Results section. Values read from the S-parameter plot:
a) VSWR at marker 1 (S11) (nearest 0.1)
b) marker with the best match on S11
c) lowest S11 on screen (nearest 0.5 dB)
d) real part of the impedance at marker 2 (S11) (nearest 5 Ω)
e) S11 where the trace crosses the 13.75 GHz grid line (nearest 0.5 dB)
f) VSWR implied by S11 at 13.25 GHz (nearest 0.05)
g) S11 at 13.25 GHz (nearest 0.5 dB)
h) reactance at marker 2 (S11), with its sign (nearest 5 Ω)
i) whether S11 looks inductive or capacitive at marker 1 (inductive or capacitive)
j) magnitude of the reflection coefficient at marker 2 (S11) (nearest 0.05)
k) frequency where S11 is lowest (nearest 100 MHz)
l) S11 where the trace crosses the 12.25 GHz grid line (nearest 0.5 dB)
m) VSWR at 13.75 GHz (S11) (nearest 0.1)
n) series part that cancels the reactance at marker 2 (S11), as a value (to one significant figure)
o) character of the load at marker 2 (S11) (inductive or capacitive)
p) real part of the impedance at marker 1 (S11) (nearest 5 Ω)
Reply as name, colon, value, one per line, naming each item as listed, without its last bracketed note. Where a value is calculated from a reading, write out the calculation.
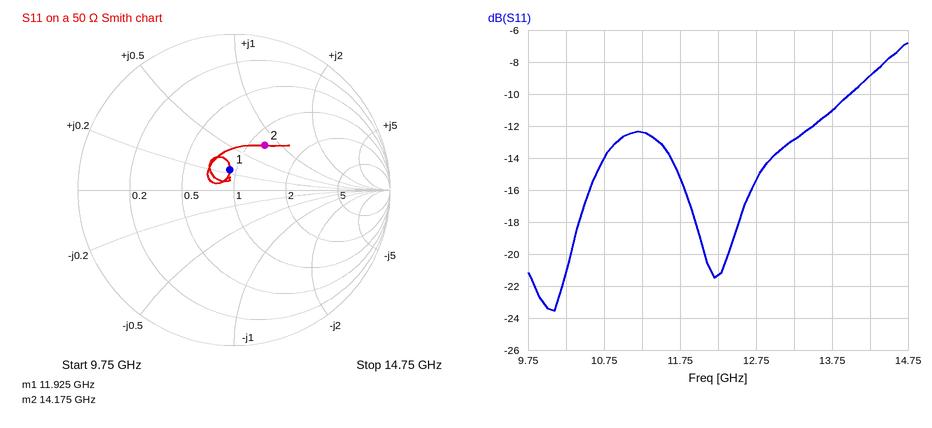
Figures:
VSWR at marker 1 (S11): 1.3
marker with the best match on S11: marker 1
lowest S11 on screen: -23.5 dB
real part of the impedance at marker 2 (S11): 60 Ω
S11 where the trace crosses the 13.75 GHz grid line: -11.0 dB
VSWR implied by S11 at 13.25 GHz: |Γ| = 10^(-13/20) = 0.2239; VSWR = (1 + 0.2239)/(1 − 0.2239) ≈ 1.58, so 1.60 to the nearest 0.05
S11 at 13.25 GHz: -13.0 dB
reactance at marker 2 (S11), with its sign: +40 Ω
whether S11 looks inductive or capacitive at marker 1: inductive
magnitude of the reflection coefficient at marker 2 (S11): 0.35
frequency where S11 is lowest: 10.1 GHz
S11 where the trace crosses the 12.25 GHz grid line: -21.5 dB
VSWR at 13.75 GHz (S11): |Γ| = 10^(-11/20) = 0.2818; VSWR = (1 + 0.2818)/(1 − 0.2818) ≈ 1.8
series part that cancels the reactance at marker 2 (S11), as a value: C = 1/(2π × 14.175 GHz × 40 Ω) ≈ 281 fF, so 300 fF to one significant figure
character of the load at marker 2 (S11): inductive
real part of the impedance at marker 1 (S11): 45 Ω
